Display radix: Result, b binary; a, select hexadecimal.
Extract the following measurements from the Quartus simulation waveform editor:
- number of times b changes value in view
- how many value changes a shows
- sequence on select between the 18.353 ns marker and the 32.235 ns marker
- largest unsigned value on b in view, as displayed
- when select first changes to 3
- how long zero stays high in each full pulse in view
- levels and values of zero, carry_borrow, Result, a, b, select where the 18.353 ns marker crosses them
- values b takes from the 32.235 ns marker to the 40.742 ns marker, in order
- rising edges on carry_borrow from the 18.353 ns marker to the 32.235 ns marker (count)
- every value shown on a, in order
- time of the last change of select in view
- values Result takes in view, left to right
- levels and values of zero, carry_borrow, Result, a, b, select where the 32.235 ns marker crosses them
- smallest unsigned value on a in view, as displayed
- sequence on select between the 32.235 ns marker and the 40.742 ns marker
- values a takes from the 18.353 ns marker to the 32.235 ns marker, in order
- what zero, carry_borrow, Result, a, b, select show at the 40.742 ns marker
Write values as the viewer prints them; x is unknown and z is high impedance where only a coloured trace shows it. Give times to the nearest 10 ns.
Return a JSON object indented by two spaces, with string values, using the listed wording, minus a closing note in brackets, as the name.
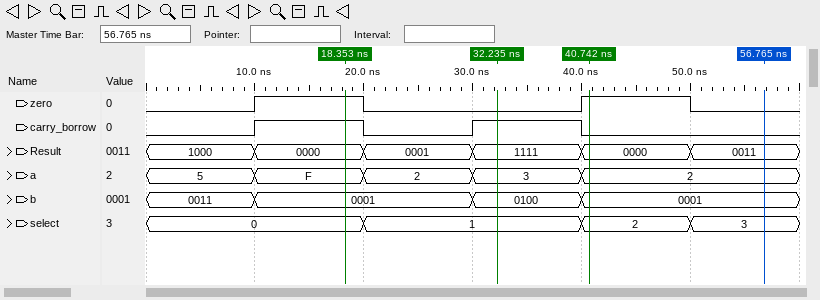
{
  "number of times b changes value in view": "3",
  "how many value changes a shows": "4",
  "sequence on select between the 18.353 ns marker and the 32.235 ns marker": "0, 1",
  "largest unsigned value on b in view, as displayed": "0100",
  "when select first changes to 3": "50 ns",
  "how long zero stays high in each full pulse in view": "10 ns, 10 ns",
  "levels and values of zero, carry_borrow, Result, a, b, select where the 18.353 ns marker crosses them": "zero=1, carry_borrow=1, Result=0000, a=F, b=0001, select=0",
  "values b takes from the 32.235 ns marker to the 40.742 ns marker, in order": "0100, 0001",
  "rising edges on carry_borrow from the 18.353 ns marker to the 32.235 ns marker": "1",
  "every value shown on a, in order": "5, F, 2, 3, 2",
  "time of the last change of select in view": "50 ns",
  "values Result takes in view, left to right": "1000, 0000, 0001, 1111, 0000, 0011",
  "levels and values of zero, carry_borrow, Result, a, b, select where the 32.235 ns marker crosses them": "zero=0, carry_borrow=1, Result=1111, a=3, b=0100, select=1",
  "smallest unsigned value on a in view, as displayed": "2",
  "sequence on select between the 32.235 ns marker and the 40.742 ns marker": "1, 2",
  "values a takes from the 18.353 ns marker to the 32.235 ns marker, in order": "F, 2, 3",
  "what zero, carry_borrow, Result, a, b, select show at the 40.742 ns marker": "zero=1, carry_borrow=0, Result=0000, a=2, b=0001, select=2"
}
